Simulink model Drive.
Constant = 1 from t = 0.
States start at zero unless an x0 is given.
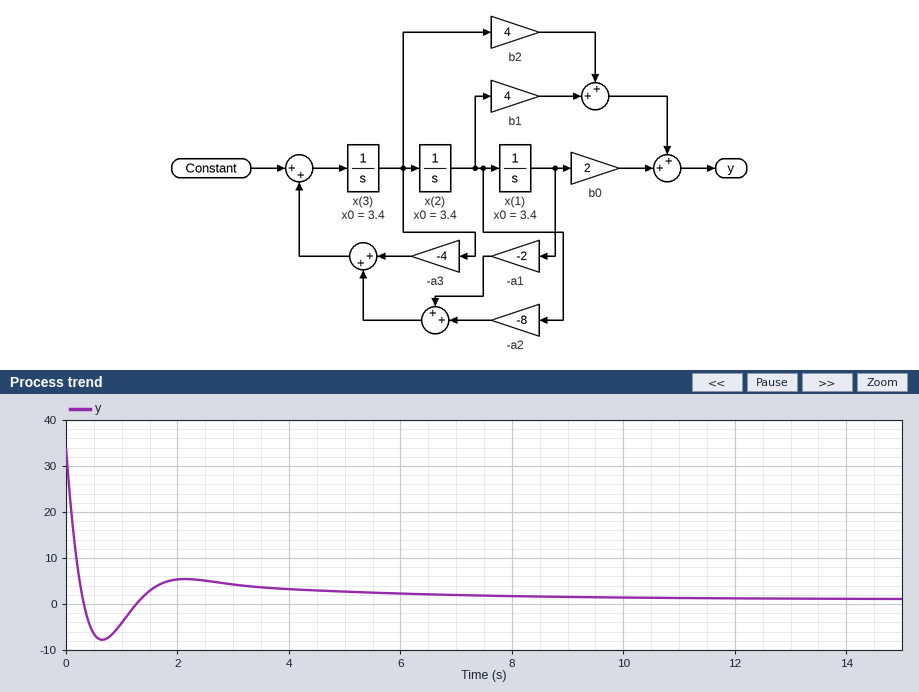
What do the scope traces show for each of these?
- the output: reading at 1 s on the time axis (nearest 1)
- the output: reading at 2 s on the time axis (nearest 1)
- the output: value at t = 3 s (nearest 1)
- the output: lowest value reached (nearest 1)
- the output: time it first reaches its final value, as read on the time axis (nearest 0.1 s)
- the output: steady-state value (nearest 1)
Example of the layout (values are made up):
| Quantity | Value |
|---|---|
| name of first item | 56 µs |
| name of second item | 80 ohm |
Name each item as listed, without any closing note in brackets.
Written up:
| Quantity | Value |
|---|---|
| the output: reading at 1 s on the time axis | -4 |
| the output: reading at 2 s on the time axis | 5 |
| the output: value at t = 3 s | 4 |
| the output: lowest value reached | -8 |
| the output: time it first reaches its final value, as read on the time axis | 0.3 s |
| the output: steady-state value | 1 |
